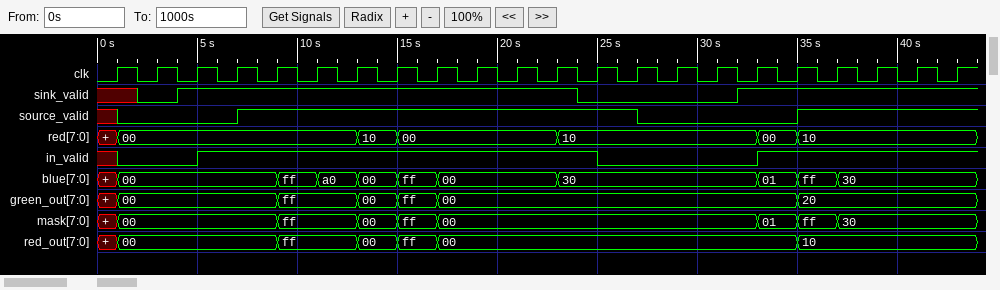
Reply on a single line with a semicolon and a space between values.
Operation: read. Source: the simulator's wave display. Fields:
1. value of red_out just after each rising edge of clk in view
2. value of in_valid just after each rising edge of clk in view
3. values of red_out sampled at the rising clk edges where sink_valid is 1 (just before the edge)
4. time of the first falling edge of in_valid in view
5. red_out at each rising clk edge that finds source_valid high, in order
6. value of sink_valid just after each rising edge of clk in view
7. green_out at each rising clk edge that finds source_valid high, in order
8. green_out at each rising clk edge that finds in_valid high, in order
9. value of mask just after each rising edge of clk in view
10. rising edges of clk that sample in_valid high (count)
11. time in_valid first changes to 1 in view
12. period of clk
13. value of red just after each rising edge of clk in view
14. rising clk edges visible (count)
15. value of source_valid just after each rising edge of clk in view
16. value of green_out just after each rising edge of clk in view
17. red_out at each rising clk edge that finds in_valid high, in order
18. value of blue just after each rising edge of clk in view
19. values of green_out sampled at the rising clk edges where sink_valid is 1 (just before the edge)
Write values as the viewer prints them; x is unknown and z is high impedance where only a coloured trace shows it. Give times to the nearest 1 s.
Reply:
00, 00, 00, 00, ff, ff, 00, ff, 00, 00, 00, 00, 00, 00, 00, 00, 00, 10, 10, 10, 10, 10; 0 0 1 1 1 1 1 1 1 1 1 1 0 0 0 0 1 1 1 1 1 1; 00, 00, 00, ff, ff, 00, ff, 00, 00, 00, 00, 00, 10, 10, 10, 10; 25 s; 00, ff, ff, 00, ff, 00, 00, 00, 00, 00, 10, 10, 10, 10; x 0 1 1 1 1 1 1 1 1 1 1 0 0 0 0 1 1 1 1 1 1; 00, ff, ff, 00, ff, 00, 00, 00, 00, 00, 20, 20, 20, 20; 00, 00, ff, ff, 00, ff, 00, 00, 00, 00, 00, 20, 20, 20, 20; 00, 00, 00, 00, ff, ff, 00, ff, 00, 00, 00, 00, 00, 00, 00, 00, 01, ff, 30, 30, 30, 30; 15; 5 s; 2 s; 00, 00, 00, 00, 00, 00, 10, 00, 00, 00, 00, 10, 10, 10, 10, 10, 00, 10, 10, 10, 10, 10; 22; 0 0 0 1 1 1 1 1 1 1 1 1 1 0 0 0 0 1 1 1 1 1; 00, 00, 00, 00, ff, ff, 00, ff, 00, 00, 00, 00, 00, 00, 00, 00, 00, 20, 20, 20, 20, 20; 00, 00, ff, ff, 00, ff, 00, 00, 00, 00, 00, 10, 10, 10, 10; 00, 00, 00, 00, ff, a0, 00, ff, 00, 00, 00, 30, 30, 30, 30, 30, 01, ff, 30, 30, 30, 30; 00, 00, 00, ff, ff, 00, ff, 00, 00, 00, 00, 00, 20, 20, 20, 20
